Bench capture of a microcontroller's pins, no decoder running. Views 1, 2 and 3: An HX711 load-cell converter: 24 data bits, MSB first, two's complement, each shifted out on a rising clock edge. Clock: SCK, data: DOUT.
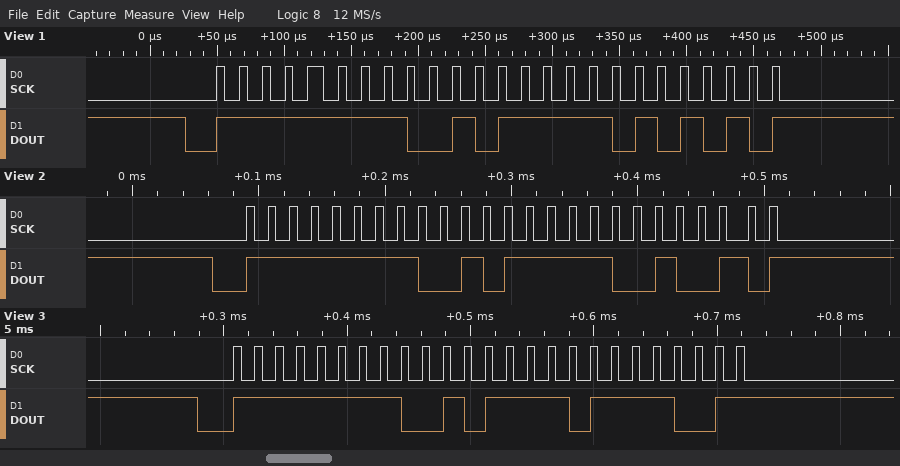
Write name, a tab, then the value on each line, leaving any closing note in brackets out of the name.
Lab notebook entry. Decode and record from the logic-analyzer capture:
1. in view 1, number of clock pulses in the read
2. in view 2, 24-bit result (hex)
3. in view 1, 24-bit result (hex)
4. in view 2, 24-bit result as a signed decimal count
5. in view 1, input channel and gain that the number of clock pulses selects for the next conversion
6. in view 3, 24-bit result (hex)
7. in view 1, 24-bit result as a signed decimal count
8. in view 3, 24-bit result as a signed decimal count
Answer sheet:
in view 1, number of clock pulses in the read	25
in view 2, 24-bit result	0xFF2F92
in view 1, 24-bit result	0xFF2FAA
in view 2, 24-bit result as a signed decimal count	-53358
in view 1, input channel and gain that the number of clock pulses selects for the next conversion	channel A, gain 128
in view 3, 24-bit result	0xFF2F79
in view 1, 24-bit result as a signed decimal count	-53334
in view 3, 24-bit result as a signed decimal count	-53383
